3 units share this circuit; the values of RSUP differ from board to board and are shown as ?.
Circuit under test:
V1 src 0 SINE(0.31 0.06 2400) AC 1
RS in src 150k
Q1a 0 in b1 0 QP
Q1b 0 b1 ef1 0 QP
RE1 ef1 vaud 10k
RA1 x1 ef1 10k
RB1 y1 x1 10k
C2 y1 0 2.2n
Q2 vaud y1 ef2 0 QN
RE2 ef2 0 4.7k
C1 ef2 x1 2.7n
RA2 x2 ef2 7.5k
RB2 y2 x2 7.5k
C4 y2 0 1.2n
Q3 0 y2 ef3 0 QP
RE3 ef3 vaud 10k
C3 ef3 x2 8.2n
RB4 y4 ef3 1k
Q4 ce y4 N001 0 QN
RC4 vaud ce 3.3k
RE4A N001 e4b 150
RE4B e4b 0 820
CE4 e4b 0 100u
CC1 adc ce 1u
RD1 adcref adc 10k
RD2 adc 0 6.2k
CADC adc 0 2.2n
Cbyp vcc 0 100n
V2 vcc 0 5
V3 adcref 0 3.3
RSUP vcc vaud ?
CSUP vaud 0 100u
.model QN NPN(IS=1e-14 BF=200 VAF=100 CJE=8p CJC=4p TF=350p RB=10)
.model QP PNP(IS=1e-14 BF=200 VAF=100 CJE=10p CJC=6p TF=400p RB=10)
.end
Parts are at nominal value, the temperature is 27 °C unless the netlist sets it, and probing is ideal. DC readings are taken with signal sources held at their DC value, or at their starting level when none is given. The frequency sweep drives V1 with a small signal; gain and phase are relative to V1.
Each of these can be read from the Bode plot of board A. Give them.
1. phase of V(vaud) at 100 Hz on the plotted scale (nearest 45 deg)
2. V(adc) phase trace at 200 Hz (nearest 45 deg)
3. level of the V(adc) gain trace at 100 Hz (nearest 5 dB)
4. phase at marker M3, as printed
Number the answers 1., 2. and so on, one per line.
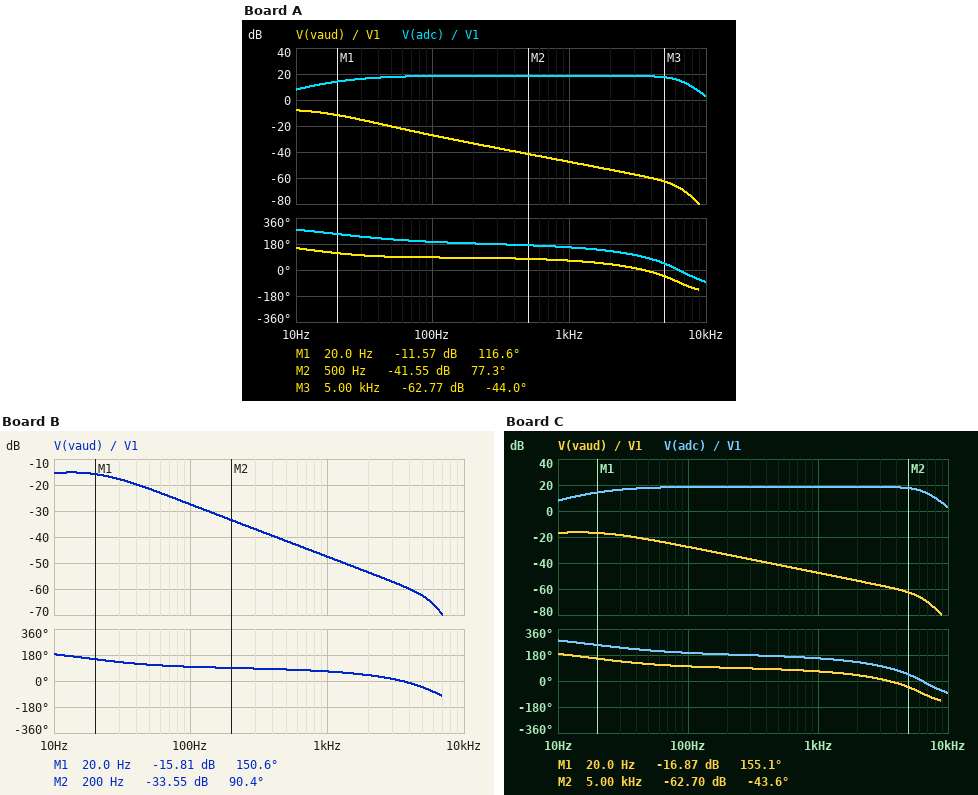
1. 90 deg
2. 180 deg
3. 20 dB
4. -44.0 deg
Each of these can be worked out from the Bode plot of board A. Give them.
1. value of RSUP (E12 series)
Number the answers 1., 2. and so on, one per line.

1. 220 Ω
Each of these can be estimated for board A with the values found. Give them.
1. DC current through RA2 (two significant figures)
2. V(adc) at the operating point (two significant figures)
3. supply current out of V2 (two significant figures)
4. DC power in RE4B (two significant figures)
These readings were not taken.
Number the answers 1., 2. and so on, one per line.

1. 1.6 µA
2. 1.3 V
3. 1.6 mA
4. 550 µW
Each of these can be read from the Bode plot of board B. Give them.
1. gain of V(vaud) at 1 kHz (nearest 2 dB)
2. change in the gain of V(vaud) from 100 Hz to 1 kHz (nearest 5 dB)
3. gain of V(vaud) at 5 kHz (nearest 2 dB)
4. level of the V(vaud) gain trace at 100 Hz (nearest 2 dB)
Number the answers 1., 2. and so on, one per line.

1. -48 dB
2. -20 dB
3. -62 dB
4. -28 dB
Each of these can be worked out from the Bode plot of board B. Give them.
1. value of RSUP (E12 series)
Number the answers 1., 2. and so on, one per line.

1. 56 Ω
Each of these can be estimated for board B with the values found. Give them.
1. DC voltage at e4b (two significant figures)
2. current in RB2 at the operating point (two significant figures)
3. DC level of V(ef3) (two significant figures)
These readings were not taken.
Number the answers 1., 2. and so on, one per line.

1. 680 mV
2. 1.7 µA
3. 1.5 V
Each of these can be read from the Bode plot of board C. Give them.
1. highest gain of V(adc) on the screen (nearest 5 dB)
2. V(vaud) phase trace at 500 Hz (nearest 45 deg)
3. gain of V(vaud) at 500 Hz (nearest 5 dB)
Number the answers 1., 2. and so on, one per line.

1. 20 dB
2. 90 deg
3. -40 dB
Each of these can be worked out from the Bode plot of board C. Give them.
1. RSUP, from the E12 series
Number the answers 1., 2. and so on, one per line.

1. 47 Ω
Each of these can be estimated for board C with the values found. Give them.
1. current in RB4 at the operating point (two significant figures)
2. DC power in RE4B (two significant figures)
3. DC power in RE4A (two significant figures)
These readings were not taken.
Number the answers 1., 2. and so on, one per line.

1. 4.1 µA
2. 560 µW
3. 100 µW
